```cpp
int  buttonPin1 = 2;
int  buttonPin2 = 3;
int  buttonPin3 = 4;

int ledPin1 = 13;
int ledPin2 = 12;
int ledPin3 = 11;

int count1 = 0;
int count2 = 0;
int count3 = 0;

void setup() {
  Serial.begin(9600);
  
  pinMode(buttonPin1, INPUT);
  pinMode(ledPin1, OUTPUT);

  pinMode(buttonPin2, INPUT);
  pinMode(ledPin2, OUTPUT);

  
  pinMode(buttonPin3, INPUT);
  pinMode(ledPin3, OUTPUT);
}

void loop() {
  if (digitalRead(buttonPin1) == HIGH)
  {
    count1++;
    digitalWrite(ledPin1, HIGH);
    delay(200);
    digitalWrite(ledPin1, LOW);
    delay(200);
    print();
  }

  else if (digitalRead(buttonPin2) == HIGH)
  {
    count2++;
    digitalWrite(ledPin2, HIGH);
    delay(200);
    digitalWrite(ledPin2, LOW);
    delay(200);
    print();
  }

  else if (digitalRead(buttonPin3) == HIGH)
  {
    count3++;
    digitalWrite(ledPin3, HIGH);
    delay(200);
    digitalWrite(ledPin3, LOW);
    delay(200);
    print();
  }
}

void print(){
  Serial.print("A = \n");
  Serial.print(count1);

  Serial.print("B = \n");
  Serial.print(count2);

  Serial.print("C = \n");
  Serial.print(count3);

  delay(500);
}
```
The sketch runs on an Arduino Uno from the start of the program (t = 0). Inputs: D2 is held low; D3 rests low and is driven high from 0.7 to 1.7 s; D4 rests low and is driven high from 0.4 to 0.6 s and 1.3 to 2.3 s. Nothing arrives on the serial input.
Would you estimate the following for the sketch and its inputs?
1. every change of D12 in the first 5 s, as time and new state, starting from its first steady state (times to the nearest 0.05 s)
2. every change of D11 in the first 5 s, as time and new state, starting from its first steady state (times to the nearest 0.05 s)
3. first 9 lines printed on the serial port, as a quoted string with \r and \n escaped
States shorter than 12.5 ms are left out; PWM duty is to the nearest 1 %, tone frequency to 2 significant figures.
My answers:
0 s low; 1.3 s high; 1.5 s low
0 s low; 0.4 s high; 0.6 s low; 2.2 s high; 2.4 s low
"A = \n0B = \n0C = \n1A = \n0B = \n1C = \n1A = \n0B = \n1C = \n"
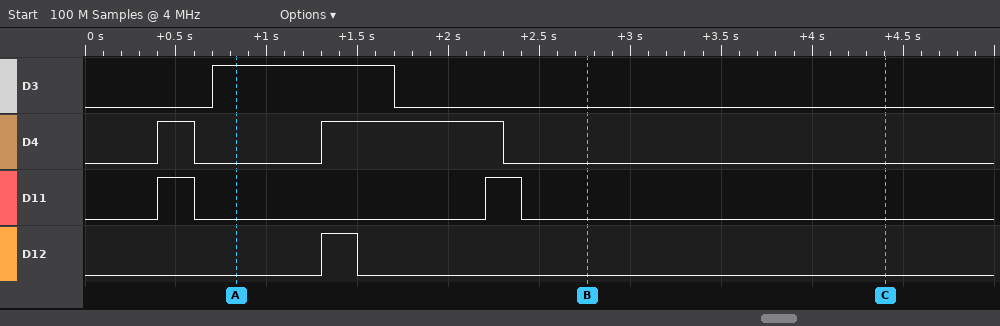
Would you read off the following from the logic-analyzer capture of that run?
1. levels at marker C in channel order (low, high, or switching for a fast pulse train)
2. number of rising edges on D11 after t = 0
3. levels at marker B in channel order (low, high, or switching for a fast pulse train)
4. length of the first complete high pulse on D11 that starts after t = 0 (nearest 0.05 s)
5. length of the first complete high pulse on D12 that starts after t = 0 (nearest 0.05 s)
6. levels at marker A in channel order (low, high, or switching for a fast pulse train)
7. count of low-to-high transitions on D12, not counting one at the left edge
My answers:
D3 low, D4 low, D11 low, D12 low
2
D3 low, D4 low, D11 low, D12 low
0.20 s
0.20 s
D3 high, D4 low, D11 low, D12 low
1
